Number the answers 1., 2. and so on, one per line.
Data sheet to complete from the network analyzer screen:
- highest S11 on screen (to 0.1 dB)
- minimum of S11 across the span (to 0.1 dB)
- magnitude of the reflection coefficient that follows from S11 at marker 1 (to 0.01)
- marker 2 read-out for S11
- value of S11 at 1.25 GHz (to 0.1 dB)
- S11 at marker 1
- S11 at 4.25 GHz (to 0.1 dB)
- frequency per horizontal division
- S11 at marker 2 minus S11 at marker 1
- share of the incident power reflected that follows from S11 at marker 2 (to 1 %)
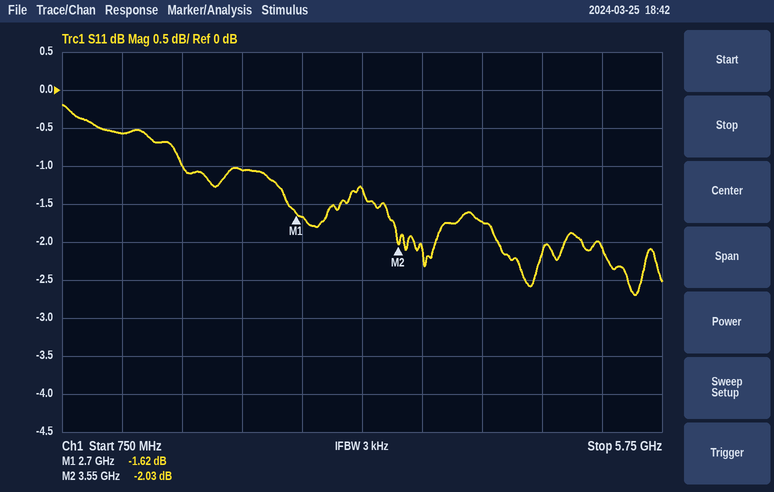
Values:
1. -0.2 dB
2. -2.7 dB
3. 0.83
4. -2.03 dB
5. -0.6 dB
6. -1.62 dB
7. -1.7 dB
8. 500 MHz
9. -0.41 dB
10. 63 %
